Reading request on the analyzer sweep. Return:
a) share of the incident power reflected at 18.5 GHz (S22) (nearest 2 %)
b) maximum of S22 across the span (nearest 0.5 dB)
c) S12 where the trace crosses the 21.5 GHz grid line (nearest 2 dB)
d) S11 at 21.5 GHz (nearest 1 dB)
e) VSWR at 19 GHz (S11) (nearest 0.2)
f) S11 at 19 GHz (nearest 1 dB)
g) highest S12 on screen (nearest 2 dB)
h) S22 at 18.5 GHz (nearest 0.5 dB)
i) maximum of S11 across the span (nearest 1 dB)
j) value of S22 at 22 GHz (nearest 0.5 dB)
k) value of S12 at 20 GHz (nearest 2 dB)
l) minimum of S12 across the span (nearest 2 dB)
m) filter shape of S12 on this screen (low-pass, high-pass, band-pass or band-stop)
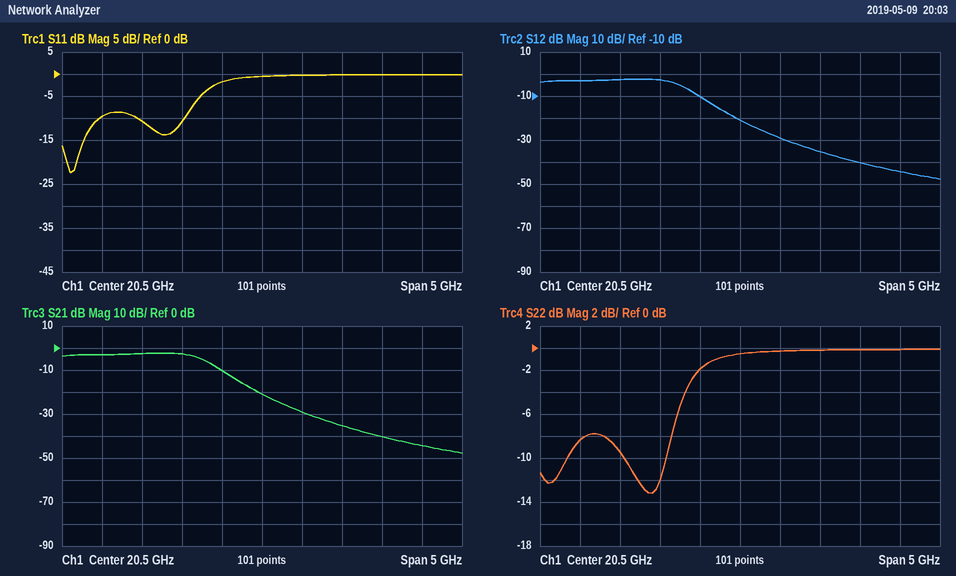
14 %
0.0 dB
-36 dB
0 dB
1.8
-11 dB
-2 dB
-8.5 dB
0 dB
0.0 dB
-10 dB
-48 dB
low-pass
